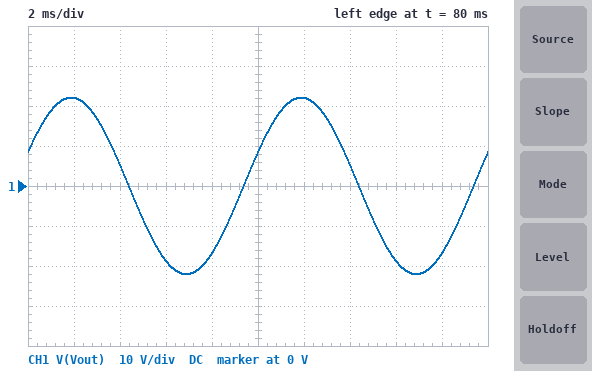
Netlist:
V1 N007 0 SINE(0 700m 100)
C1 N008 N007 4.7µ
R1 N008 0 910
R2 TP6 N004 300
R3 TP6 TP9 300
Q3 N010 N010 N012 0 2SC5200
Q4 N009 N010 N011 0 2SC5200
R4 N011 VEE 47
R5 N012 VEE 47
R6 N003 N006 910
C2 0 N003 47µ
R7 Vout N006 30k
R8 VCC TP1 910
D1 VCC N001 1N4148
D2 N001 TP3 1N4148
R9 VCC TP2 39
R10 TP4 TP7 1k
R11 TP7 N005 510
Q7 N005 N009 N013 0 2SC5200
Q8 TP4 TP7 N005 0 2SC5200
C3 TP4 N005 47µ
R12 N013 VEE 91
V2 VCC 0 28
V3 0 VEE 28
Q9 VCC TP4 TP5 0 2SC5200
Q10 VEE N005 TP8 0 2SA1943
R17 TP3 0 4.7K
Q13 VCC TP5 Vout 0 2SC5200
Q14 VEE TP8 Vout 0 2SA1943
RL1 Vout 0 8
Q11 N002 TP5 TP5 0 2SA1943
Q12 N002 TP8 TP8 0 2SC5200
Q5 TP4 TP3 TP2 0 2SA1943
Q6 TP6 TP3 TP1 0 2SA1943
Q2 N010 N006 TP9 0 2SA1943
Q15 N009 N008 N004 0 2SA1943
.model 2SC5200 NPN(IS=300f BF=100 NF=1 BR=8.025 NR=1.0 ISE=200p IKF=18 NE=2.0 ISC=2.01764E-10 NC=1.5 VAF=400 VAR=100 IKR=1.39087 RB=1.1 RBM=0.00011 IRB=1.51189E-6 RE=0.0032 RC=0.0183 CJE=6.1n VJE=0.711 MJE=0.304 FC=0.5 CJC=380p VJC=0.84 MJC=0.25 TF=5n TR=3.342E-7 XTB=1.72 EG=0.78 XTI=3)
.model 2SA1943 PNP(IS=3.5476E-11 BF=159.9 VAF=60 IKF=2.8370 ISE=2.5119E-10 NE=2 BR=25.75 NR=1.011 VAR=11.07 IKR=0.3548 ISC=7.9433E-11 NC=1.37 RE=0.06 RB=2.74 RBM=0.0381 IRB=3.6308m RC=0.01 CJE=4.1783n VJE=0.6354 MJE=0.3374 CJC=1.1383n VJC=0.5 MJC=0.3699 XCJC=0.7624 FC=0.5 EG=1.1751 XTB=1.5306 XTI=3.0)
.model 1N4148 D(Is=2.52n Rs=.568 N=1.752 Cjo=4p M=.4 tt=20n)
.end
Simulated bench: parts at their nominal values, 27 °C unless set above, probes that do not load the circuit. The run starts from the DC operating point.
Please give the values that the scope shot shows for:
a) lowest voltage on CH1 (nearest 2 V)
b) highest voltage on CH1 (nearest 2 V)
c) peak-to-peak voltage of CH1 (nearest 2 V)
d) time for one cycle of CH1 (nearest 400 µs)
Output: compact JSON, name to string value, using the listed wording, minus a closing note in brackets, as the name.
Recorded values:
{"lowest voltage on CH1": "-22 V", "highest voltage on CH1": "22 V", "peak-to-peak voltage of CH1": "44 V", "time for one cycle of CH1": "10.0 ms"}
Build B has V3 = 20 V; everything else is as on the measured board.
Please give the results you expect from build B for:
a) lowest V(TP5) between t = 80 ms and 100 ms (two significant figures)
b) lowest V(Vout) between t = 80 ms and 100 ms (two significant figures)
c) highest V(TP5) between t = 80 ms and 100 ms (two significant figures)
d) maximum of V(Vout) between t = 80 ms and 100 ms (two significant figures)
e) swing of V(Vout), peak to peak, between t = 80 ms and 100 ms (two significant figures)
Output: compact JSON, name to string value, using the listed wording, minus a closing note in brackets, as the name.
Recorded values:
{"lowest V(TP5) between t = 80 ms and 100 ms": "-16 V", "lowest V(Vout) between t = 80 ms and 100 ms": "-17 V", "highest V(TP5) between t = 80 ms and 100 ms": "22 V", "maximum of V(Vout) between t = 80 ms and 100 ms": "21 V", "swing of V(Vout), peak to peak, between t = 80 ms and 100 ms": "38 V"}
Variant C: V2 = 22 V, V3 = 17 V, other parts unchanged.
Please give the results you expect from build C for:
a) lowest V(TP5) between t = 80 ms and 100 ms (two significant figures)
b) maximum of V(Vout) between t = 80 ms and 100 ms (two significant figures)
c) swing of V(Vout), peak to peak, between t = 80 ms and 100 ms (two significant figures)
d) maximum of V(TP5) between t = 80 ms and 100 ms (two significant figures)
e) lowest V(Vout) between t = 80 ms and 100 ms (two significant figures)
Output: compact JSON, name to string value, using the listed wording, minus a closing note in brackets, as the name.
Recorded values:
{"lowest V(TP5) between t = 80 ms and 100 ms": "-13 V", "maximum of V(Vout) between t = 80 ms and 100 ms": "20 V", "swing of V(Vout), peak to peak, between t = 80 ms and 100 ms": "34 V", "maximum of V(TP5) between t = 80 ms and 100 ms": "21 V", "lowest V(Vout) between t = 80 ms and 100 ms": "-14 V"}
